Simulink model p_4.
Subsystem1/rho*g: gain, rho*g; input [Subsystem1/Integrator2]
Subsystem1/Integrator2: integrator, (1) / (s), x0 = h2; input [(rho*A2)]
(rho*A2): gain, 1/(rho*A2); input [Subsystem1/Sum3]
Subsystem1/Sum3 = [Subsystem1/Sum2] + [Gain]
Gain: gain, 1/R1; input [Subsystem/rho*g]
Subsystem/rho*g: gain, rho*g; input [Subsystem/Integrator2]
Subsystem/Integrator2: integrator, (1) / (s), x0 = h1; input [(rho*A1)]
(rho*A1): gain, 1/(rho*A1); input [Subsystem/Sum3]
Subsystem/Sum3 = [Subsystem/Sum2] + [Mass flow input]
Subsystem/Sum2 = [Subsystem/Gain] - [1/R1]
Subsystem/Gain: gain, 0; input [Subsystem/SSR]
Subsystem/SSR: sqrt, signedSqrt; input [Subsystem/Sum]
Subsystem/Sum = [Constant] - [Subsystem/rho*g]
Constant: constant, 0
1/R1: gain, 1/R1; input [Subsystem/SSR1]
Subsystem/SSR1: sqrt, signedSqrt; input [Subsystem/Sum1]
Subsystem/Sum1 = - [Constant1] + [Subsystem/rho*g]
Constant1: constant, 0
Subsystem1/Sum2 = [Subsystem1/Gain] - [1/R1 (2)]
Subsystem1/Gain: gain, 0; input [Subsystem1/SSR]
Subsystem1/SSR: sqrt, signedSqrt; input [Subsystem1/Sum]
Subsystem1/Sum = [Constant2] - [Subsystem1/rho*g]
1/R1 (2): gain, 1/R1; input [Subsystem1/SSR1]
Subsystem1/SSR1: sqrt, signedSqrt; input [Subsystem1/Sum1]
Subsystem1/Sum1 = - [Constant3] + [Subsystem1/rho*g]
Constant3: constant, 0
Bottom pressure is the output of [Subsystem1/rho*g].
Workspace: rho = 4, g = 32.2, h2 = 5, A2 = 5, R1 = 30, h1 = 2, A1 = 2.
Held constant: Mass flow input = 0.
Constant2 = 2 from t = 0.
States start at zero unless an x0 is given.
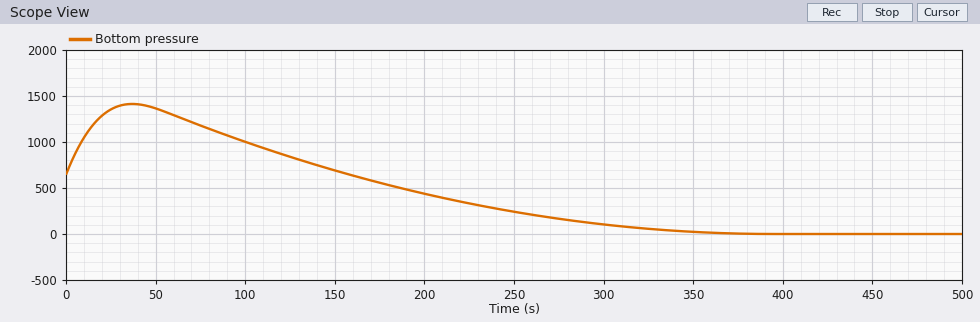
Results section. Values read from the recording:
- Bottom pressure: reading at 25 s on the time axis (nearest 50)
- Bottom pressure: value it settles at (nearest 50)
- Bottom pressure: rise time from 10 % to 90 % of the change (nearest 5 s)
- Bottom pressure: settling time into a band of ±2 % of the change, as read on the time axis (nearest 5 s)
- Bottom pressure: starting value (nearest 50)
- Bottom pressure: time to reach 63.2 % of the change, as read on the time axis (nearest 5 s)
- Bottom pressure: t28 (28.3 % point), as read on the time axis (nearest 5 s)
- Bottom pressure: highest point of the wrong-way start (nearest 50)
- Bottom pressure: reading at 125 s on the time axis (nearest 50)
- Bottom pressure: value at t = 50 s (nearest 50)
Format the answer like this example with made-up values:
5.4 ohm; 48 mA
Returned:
1350; 0; 150 s; 360 s; 650; 250 s; 195 s; 1400; 850; 1350
